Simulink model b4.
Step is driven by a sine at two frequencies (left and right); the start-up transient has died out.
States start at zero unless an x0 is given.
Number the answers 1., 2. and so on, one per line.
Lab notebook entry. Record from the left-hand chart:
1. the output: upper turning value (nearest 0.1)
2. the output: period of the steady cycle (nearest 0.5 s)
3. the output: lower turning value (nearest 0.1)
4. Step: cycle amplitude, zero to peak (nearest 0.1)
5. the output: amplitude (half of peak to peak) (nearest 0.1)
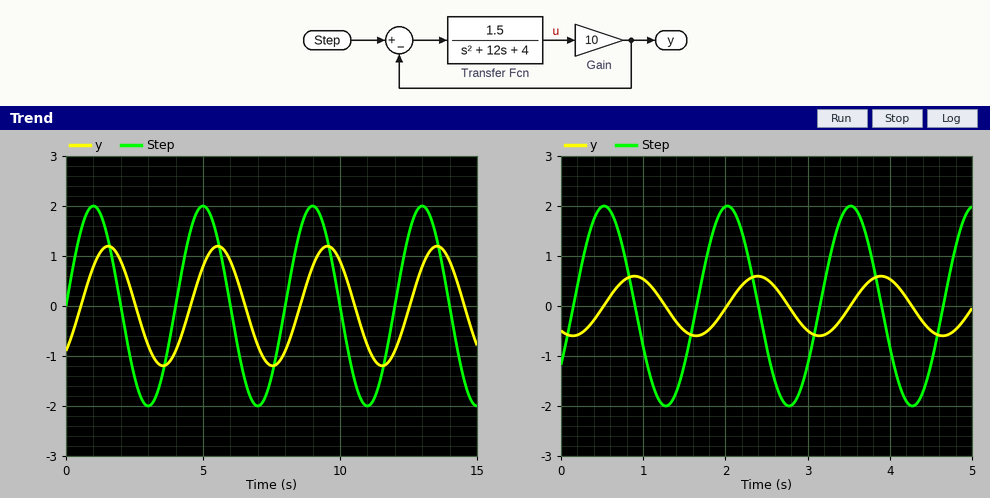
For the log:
1. 1.2
2. 4.0 s
3. -1.2
4. 2.0
5. 1.2
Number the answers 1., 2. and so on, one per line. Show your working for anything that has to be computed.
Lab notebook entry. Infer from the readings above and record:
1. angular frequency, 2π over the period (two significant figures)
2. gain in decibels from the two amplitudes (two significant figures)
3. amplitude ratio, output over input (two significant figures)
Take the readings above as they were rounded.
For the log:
1. 2π / 4 = 1.6 rad/s
2. 20 log10(1.2 / 2) = -4.4 dB
3. 1.2 / 2 = 0.60
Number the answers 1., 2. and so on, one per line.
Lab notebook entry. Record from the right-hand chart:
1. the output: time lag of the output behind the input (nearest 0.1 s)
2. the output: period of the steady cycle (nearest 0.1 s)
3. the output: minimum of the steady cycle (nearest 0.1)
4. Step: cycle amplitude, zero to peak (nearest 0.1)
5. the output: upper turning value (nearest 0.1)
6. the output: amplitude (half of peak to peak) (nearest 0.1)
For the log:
1. 0.4 s
2. 1.5 s
3. -0.6
4. 2.0
5. 0.6
6. 0.6
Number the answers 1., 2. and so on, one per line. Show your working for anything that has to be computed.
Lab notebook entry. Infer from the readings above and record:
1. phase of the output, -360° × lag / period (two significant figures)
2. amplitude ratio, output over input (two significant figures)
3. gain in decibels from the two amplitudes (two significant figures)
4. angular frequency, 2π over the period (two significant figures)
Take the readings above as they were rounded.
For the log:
1. -360 × 0.4 / 1.5 = -96°
2. 0.6 / 2 = 0.30
3. 20 log10(0.6 / 2) = -10 dB
4. 2π / 1.5 = 4.2 rad/s
